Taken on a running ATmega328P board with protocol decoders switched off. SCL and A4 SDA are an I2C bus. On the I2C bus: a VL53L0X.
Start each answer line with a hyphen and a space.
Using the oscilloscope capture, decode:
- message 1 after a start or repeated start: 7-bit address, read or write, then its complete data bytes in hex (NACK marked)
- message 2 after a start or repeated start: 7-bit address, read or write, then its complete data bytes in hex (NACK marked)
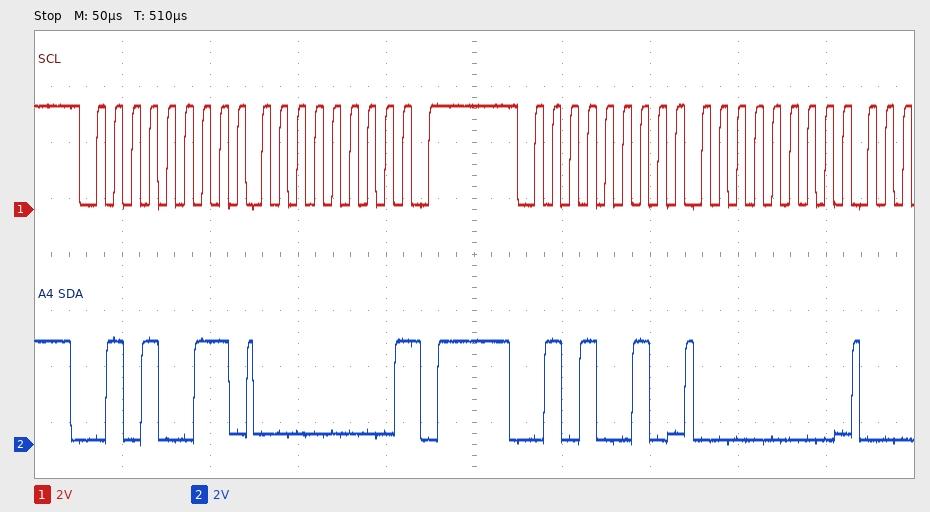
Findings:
- 0x29 read: 00 NACK
- 0x29 write: 00
